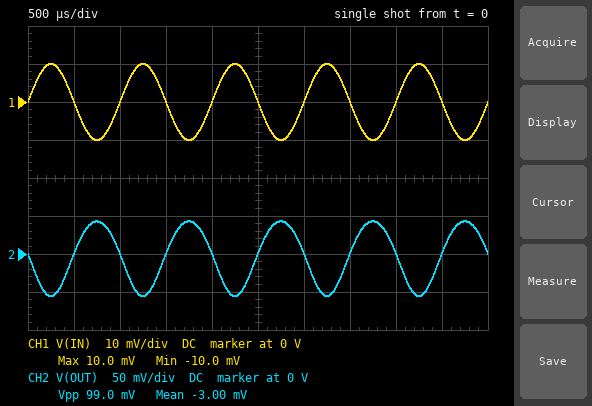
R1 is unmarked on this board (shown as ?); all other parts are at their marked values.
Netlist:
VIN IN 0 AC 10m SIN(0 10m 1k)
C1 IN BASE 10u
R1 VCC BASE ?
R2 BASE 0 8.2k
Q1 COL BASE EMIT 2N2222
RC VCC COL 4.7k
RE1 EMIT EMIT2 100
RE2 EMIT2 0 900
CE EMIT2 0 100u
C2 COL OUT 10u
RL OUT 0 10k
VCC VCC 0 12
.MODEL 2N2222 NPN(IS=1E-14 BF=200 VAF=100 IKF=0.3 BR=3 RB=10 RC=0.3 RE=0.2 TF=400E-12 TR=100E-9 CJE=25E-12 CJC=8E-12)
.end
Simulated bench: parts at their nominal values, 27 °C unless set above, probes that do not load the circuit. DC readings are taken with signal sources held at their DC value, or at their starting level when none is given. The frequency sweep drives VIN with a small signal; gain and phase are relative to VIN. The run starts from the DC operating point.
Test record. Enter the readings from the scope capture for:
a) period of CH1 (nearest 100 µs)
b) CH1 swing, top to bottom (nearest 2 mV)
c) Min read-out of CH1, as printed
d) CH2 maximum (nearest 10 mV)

1.0 ms
20 mV
-10.0 mV
40 mV
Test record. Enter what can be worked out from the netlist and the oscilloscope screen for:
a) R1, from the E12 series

150 kΩ
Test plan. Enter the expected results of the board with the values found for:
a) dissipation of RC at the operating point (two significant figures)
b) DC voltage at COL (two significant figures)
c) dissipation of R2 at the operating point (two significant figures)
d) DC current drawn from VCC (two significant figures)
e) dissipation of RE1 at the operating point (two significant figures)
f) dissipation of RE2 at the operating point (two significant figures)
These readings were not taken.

10 µW
12 V
47 µW
120 µA
220 nW
2.0 µW
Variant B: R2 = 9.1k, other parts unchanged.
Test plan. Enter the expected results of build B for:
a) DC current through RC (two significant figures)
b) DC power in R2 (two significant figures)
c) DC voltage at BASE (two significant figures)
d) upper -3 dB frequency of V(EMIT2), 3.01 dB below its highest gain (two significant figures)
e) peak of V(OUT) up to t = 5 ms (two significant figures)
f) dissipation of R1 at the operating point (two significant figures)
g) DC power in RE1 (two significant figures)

92 µA
51 µW
680 mV
9.2 Hz
76 mV
850 µW
850 nW
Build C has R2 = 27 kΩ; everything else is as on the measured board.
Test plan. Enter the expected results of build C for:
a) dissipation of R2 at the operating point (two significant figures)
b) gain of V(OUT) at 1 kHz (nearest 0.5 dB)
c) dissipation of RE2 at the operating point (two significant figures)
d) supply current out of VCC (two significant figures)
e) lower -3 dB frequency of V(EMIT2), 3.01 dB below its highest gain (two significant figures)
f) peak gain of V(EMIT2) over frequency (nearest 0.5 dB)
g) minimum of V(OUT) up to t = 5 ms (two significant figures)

110 µW
28.0 dB
1.0 mW
1.1 mA
680 mHz
-2.0 dB
-250 mV
